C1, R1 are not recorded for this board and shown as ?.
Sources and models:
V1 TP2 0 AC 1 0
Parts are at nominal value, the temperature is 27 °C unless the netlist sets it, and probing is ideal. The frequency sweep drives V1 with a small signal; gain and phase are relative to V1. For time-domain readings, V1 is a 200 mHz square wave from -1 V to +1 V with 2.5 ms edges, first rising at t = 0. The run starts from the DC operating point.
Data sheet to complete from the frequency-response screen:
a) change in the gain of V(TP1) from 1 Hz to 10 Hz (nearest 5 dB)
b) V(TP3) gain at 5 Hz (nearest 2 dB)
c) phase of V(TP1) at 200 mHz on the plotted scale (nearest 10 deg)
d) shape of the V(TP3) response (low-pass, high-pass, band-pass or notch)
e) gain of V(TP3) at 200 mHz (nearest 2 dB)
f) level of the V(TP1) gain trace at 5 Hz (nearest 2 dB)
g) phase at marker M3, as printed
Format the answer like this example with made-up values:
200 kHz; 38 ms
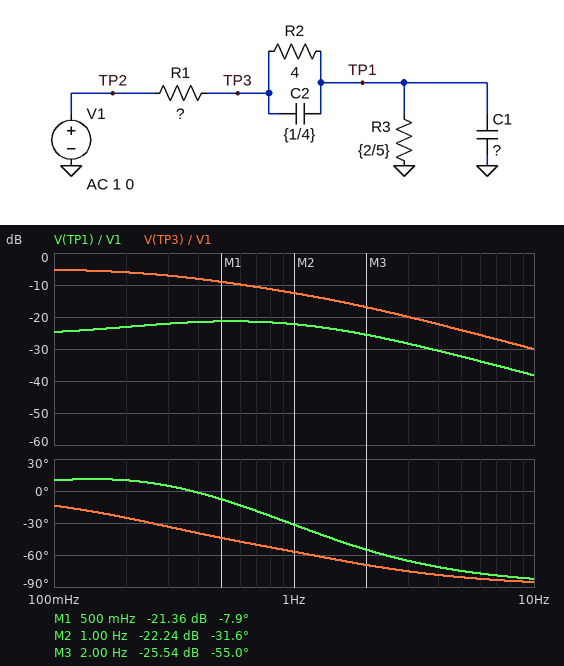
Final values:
-15 dB; -24 dB; 10 deg; low-pass; -6 dB; -32 dB; -55.0 deg
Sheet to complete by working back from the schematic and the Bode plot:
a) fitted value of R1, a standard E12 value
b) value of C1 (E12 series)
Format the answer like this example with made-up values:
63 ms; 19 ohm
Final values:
3.3 Ω; 390 mF
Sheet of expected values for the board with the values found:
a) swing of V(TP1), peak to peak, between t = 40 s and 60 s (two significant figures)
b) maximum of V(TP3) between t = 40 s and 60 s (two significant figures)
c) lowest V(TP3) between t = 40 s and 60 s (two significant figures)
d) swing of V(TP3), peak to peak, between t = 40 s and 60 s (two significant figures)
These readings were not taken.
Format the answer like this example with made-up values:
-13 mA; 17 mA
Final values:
210 mV; 570 mV; -570 mV; 1.1 V
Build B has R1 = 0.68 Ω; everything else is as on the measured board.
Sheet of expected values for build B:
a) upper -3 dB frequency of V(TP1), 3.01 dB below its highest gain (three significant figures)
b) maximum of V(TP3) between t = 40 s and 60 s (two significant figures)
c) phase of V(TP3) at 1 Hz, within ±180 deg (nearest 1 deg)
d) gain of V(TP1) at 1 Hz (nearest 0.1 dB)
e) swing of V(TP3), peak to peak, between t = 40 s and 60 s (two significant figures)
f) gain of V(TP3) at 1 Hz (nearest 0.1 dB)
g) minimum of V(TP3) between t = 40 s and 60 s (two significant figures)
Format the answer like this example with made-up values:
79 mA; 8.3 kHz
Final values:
3.06 Hz; 870 mV; -30 deg; -13.0 dB; 1.7 V; -3.3 dB; -870 mV
